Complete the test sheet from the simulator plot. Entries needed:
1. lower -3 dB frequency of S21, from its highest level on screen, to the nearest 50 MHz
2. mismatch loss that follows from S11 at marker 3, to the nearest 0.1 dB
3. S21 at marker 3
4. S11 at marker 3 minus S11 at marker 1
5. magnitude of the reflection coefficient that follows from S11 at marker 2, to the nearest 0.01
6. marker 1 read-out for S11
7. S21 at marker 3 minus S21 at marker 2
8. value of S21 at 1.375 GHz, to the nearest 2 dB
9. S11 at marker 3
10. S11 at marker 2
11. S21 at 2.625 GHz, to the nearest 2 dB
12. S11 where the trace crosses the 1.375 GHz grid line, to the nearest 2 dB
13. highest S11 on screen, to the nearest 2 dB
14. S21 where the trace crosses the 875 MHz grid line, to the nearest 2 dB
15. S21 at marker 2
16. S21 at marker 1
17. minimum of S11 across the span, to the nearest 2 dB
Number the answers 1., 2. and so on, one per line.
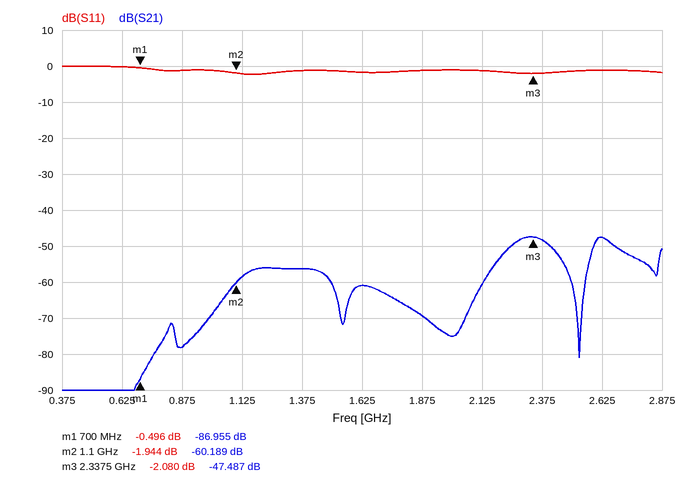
1. 2.25 GHz
2. 4.2 dB
3. -47.487 dB
4. -1.584 dB
5. 0.80
6. -0.496 dB
7. 12.702 dB
8. -56 dB
9. -2.080 dB
10. -1.944 dB
11. -48 dB
12. -2 dB
13. 0 dB
14. -78 dB
15. -60.189 dB
16. -86.955 dB
17. -2 dB
